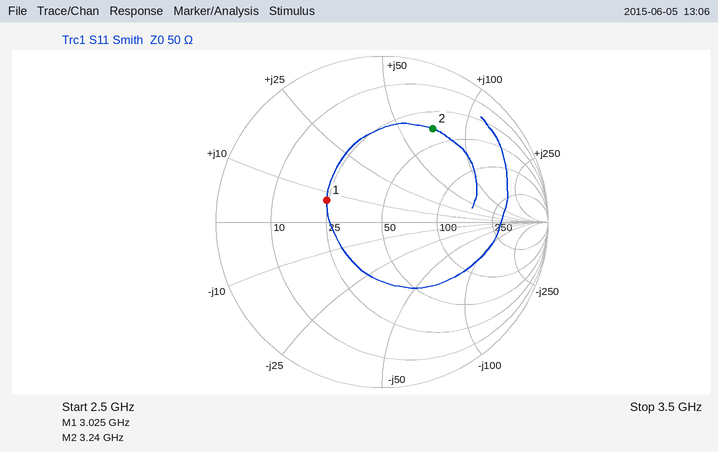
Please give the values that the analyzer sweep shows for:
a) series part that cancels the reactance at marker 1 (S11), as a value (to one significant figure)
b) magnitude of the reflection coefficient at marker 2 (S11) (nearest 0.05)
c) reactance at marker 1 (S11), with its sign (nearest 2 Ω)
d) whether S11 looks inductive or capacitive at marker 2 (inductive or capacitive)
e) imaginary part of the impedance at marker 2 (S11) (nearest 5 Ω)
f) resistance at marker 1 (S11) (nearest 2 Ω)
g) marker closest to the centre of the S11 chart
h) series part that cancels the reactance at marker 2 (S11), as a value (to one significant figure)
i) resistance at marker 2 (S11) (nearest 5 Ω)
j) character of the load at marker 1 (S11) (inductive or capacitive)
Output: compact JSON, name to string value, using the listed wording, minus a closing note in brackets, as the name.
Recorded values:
{"series part that cancels the reactance at marker 1 (S11), as a value": "7 pF", "magnitude of the reflection coefficient at marker 2 (S11)": "0.65", "reactance at marker 1 (S11), with its sign": "+8 Ω", "whether S11 looks inductive or capacitive at marker 2": "inductive", "imaginary part of the impedance at marker 2 (S11)": "+70 Ω", "resistance at marker 1 (S11)": "24 Ω", "marker closest to the centre of the S11 chart": "marker 1", "series part that cancels the reactance at marker 2 (S11), as a value": "700 fF", "resistance at marker 2 (S11)": "35 Ω", "character of the load at marker 1 (S11)": "inductive"}
